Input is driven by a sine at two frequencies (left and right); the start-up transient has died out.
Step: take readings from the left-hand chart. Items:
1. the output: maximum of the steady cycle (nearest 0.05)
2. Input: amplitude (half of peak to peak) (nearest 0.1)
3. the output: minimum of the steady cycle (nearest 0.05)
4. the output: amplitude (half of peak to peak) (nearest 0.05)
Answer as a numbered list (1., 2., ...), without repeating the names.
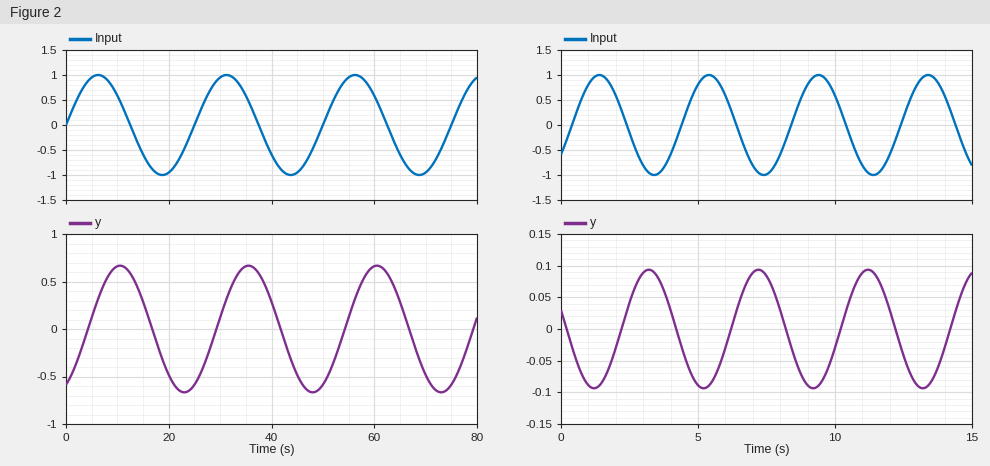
1. 0.65
2. 1.0
3. -0.65
4. 0.65
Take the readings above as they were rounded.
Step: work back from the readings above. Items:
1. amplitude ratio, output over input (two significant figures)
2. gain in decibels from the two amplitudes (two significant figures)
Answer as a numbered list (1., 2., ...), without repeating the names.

1. 0.65
2. -3.7 dB
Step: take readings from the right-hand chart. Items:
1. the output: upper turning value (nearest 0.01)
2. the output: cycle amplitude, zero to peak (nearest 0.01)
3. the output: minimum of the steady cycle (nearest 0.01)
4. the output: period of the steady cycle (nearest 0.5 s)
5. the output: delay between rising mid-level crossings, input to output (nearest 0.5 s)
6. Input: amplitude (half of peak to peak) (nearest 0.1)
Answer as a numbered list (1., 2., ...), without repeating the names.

1. 0.09
2. 0.09
3. -0.09
4. 4.0 s
5. 2.0 s
6. 1.0
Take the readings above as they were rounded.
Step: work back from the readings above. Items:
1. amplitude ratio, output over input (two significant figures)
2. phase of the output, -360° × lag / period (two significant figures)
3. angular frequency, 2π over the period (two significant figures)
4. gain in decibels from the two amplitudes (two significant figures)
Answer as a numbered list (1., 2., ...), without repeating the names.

1. 0.090
2. -180°
3. 1.6 rad/s
4. -21 dB
